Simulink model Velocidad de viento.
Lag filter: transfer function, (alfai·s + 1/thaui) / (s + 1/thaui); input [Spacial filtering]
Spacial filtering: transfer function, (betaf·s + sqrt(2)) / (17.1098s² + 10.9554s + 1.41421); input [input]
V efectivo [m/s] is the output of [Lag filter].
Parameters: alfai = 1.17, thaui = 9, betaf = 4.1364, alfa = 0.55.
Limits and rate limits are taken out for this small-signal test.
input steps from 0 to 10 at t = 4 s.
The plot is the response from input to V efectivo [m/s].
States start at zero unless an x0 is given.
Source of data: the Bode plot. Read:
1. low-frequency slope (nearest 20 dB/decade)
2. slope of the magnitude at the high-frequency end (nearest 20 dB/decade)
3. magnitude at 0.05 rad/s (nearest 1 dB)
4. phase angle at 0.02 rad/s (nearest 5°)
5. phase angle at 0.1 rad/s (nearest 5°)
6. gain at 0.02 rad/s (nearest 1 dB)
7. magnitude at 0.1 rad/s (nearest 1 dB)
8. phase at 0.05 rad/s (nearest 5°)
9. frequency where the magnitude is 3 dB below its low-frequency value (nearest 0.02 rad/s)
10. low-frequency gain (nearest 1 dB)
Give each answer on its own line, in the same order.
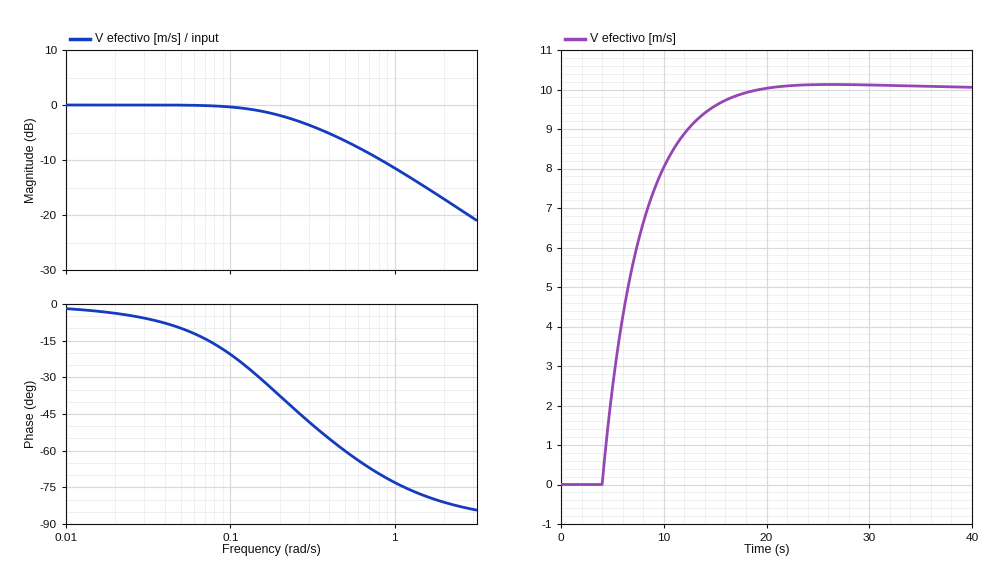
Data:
0 dB/decade
-20 dB/decade
0 dB
-5°
-20°
0 dB
0 dB
-10°
0.26 rad/s
0 dB
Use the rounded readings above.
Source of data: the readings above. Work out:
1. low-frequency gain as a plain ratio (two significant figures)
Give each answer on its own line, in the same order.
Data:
1.0
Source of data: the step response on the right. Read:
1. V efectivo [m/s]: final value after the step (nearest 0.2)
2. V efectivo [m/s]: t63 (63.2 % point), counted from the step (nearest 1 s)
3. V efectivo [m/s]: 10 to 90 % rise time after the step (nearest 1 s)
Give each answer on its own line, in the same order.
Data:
10.0
4 s
8 s
